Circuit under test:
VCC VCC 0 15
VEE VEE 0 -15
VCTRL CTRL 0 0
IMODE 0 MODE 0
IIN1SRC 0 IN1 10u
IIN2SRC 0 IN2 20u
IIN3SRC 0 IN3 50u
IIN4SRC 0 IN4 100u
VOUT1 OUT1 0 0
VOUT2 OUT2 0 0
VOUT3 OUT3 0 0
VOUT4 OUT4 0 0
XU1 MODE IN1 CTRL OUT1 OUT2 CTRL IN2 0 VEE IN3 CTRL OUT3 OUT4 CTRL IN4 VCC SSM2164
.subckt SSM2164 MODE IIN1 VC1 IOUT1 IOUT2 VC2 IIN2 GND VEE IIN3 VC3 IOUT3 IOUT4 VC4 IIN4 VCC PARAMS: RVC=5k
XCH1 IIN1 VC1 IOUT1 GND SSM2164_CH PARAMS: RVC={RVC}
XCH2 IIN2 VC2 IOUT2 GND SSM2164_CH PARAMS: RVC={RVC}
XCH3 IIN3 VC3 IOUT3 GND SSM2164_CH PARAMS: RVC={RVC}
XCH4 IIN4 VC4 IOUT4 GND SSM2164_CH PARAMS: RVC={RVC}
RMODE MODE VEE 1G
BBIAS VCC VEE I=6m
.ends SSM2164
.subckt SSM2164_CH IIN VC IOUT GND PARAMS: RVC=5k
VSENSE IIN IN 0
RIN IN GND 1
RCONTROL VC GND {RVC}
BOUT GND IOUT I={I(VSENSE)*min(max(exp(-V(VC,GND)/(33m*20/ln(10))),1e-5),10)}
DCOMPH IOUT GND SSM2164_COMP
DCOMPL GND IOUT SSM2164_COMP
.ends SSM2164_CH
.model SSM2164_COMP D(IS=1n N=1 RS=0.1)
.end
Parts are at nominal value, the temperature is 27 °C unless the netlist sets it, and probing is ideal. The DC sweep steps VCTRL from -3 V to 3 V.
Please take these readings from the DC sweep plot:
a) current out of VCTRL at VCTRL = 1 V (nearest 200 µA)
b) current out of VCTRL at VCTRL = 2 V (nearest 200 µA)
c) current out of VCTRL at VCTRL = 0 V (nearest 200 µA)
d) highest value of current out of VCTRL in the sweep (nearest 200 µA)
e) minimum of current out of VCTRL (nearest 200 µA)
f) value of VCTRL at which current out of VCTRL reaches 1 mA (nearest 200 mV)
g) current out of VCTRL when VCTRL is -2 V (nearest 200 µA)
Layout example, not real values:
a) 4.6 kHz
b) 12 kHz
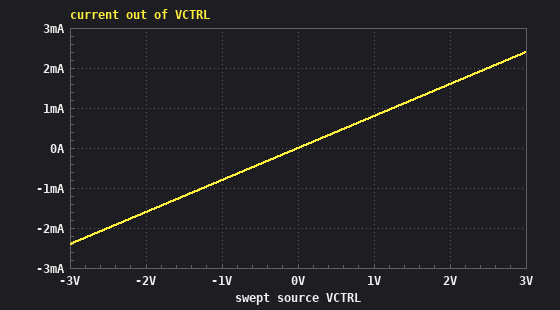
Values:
a) 800 µA
b) 1.6 mA
c) 0 A
d) 2.4 mA
e) -2.4 mA
f) 1.2 V
g) -1.6 mA
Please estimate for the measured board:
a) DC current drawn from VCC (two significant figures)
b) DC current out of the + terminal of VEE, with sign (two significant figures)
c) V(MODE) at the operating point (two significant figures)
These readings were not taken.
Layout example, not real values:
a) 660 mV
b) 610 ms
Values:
a) 6.0 mA
b) -6.0 mA
c) -15 V
